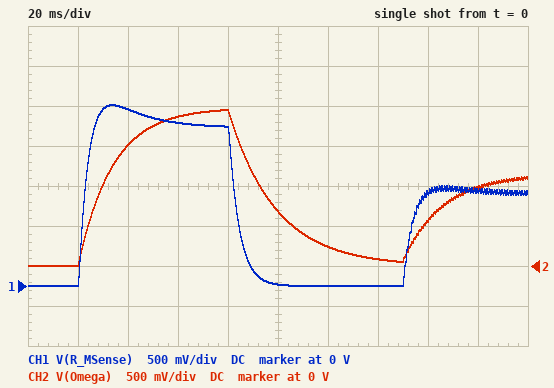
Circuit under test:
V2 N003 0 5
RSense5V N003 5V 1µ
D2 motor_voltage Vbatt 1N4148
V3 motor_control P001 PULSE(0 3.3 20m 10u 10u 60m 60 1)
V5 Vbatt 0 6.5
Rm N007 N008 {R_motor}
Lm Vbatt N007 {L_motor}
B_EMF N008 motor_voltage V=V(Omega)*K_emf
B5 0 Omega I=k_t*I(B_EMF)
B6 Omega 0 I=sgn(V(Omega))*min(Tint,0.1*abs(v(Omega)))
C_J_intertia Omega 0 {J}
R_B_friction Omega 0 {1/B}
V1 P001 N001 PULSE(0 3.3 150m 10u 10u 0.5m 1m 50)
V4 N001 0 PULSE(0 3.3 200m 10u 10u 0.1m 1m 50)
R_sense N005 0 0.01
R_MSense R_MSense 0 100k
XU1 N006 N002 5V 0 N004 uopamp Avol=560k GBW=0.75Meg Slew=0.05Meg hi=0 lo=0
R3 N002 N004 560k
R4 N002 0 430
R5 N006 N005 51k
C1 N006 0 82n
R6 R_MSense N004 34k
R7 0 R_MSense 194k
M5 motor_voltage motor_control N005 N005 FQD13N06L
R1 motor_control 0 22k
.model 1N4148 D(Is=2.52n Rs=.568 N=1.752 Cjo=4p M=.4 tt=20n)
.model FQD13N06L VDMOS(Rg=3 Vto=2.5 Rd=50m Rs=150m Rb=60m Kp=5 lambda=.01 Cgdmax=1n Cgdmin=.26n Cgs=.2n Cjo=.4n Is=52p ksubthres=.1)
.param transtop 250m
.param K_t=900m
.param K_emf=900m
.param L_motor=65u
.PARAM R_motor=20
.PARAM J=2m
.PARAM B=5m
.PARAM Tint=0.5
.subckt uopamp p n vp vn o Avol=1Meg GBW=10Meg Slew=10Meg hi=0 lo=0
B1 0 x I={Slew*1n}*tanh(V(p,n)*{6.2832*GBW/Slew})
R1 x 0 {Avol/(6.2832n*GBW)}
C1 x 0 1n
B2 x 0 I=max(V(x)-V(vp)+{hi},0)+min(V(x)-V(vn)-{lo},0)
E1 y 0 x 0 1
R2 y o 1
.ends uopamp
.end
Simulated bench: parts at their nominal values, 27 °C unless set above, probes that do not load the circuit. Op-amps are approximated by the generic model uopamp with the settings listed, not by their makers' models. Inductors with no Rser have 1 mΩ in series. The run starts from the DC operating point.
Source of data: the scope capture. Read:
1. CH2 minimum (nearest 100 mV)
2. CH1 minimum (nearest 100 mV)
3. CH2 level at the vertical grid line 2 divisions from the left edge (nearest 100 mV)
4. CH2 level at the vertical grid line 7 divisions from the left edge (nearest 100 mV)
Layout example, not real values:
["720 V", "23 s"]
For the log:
["0 V", "0 V", "1.5 V", "100 mV"]
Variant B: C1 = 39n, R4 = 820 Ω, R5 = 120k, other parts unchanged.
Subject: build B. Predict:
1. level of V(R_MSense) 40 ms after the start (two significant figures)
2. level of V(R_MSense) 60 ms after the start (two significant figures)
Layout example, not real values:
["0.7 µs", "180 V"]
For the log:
["1.2 V", "1.1 V"]
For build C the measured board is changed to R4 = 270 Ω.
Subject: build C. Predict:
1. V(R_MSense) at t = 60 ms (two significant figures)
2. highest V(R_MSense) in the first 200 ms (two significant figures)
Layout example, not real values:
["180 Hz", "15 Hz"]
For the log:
["3.2 V", "3.3 V"]
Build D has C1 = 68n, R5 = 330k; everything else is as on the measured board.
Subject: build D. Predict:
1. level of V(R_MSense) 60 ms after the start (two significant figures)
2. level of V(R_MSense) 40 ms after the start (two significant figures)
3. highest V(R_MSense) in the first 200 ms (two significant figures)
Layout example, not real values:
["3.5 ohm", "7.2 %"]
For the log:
["1.8 V", "1.4 V", "1.9 V"]
